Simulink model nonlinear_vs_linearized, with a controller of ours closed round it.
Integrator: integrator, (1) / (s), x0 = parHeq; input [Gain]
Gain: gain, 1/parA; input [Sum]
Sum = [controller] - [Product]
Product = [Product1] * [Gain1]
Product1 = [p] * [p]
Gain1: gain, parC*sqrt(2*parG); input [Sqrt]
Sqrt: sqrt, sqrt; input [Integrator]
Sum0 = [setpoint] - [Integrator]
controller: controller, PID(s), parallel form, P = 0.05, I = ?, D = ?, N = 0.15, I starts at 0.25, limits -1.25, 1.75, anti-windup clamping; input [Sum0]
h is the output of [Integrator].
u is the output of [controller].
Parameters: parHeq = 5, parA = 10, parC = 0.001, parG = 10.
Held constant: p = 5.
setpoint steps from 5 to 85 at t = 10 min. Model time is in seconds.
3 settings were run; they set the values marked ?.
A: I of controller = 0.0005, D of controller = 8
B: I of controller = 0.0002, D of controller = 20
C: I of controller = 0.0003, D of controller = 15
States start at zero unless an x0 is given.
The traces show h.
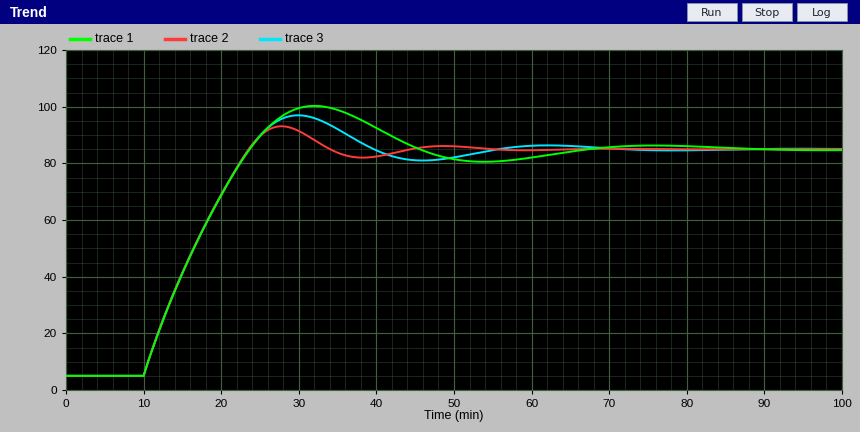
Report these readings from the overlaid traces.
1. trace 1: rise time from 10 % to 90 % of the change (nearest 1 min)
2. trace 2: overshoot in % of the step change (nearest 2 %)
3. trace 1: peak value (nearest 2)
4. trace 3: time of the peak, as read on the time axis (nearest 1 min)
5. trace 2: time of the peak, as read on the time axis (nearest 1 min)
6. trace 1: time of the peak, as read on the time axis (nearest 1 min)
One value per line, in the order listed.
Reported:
11 min
10 %
100
30 min
28 min
32 min
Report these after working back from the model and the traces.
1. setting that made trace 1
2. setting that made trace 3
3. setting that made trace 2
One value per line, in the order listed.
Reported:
B
C
A
